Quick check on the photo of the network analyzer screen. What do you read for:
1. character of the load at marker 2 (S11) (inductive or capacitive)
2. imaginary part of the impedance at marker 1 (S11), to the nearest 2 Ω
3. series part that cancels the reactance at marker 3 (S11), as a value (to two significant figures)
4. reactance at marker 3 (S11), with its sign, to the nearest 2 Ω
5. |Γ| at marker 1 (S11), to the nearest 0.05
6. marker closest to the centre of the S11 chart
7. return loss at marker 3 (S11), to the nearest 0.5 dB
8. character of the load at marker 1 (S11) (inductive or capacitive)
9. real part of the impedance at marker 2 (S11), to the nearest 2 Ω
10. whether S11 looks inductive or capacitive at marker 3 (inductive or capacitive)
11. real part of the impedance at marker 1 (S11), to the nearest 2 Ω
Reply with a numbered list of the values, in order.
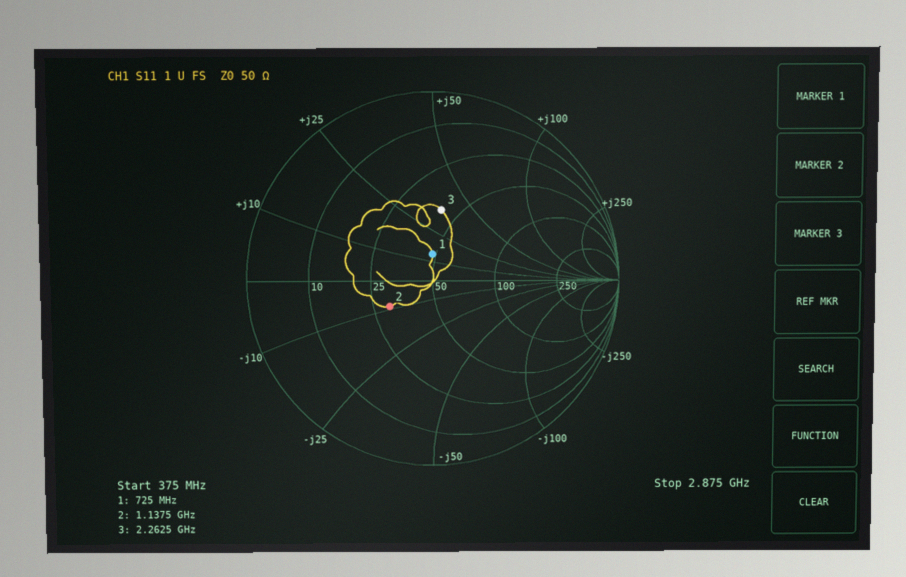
1. capacitive
2. +14 Ω
3. 2.0 pF
4. +36 Ω
5. 0.15
6. marker 1
7. 8.5 dB
8. inductive
9. 30 Ω
10. inductive
11. 48 Ω
